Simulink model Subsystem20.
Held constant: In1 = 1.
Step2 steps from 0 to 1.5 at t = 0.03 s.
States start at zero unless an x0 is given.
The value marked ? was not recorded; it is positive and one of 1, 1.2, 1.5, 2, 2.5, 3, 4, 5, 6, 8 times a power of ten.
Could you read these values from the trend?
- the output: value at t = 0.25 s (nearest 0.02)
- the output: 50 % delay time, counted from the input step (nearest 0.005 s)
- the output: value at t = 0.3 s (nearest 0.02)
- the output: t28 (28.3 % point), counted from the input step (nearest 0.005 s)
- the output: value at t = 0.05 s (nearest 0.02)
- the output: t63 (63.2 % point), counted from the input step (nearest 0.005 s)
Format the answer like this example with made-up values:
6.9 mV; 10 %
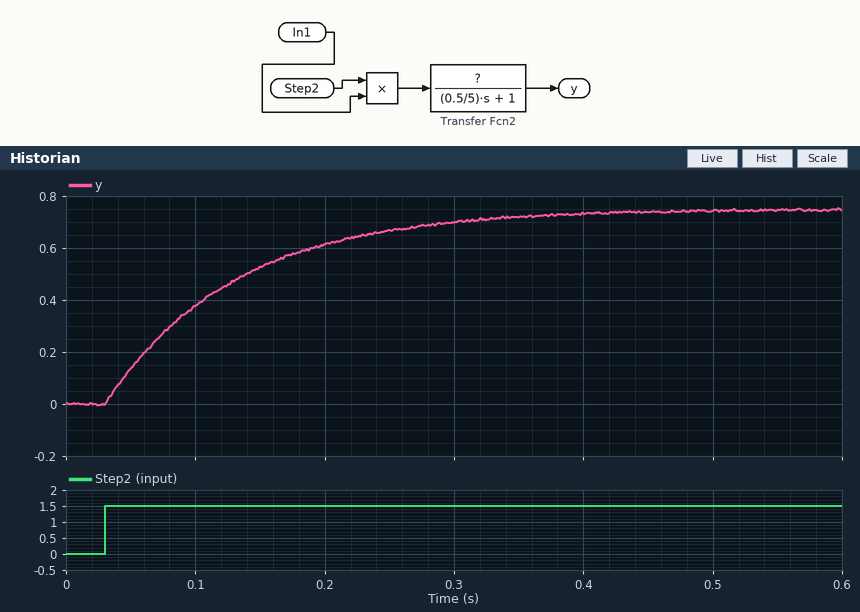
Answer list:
0.66; 0.070 s; 0.70; 0.035 s; 0.14; 0.100 s
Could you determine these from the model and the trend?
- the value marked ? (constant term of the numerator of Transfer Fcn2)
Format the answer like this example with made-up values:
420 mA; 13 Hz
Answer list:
0.5
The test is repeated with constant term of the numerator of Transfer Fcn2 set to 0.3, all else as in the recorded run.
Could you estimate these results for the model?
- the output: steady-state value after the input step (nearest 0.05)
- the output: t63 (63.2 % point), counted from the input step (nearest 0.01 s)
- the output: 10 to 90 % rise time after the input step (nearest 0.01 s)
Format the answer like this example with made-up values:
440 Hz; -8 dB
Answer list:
0.45; 0.10 s; 0.22 s
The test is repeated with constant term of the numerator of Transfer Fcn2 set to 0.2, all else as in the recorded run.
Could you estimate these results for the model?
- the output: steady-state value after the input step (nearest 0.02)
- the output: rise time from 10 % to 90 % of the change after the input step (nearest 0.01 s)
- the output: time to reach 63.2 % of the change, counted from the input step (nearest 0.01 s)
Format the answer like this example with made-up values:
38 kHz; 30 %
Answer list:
0.30; 0.22 s; 0.10 s
